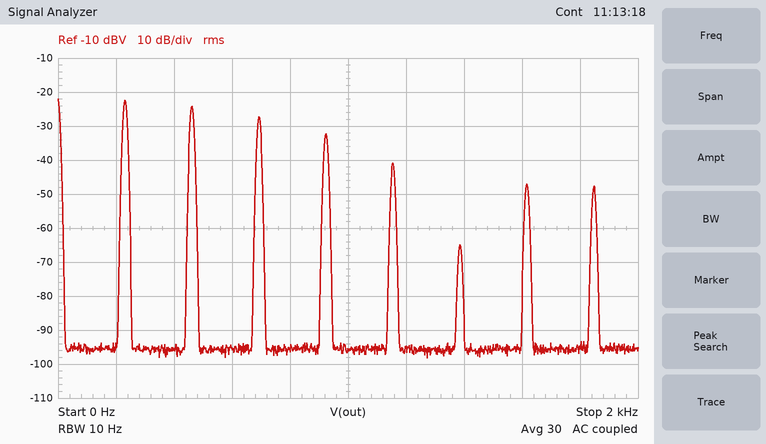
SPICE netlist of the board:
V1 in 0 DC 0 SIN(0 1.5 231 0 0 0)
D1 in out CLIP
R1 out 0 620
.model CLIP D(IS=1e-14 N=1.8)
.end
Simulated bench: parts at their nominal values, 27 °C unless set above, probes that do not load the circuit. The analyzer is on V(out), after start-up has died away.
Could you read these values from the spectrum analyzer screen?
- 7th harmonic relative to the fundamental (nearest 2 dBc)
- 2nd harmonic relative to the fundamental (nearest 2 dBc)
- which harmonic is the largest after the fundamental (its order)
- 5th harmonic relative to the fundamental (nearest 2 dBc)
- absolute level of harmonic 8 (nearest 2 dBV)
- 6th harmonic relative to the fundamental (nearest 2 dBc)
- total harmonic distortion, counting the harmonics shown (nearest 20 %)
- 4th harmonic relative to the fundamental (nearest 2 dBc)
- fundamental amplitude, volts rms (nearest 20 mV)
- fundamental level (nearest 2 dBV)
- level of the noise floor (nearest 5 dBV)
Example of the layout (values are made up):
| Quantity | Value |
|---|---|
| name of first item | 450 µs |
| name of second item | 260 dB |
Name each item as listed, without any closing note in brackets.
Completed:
| Quantity | Value |
|---|---|
| 7th harmonic relative to the fundamental | -24 dBc |
| 2nd harmonic relative to the fundamental | -2 dBc |
| which harmonic is the largest after the fundamental | 2 |
| 5th harmonic relative to the fundamental | -18 dBc |
| absolute level of harmonic 8 | -48 dBV |
| 6th harmonic relative to the fundamental | -42 dBc |
| total harmonic distortion, counting the harmonics shown | 100 % |
| 4th harmonic relative to the fundamental | -10 dBc |
| fundamental amplitude, volts rms | 80 mV |
| fundamental level | -22 dBV |
| level of the noise floor | -95 dBV |
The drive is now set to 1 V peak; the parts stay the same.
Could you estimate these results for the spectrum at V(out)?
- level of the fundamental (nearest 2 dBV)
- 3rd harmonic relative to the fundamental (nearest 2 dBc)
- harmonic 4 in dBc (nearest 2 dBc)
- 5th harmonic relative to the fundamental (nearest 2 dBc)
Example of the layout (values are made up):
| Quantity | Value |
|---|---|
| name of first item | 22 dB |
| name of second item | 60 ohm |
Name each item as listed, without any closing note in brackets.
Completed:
| Quantity | Value |
|---|---|
| level of the fundamental | -58 dBV |
| 3rd harmonic relative to the fundamental | -2 dBc |
| harmonic 4 in dBc | -4 dBc |
| 5th harmonic relative to the fundamental | -6 dBc |
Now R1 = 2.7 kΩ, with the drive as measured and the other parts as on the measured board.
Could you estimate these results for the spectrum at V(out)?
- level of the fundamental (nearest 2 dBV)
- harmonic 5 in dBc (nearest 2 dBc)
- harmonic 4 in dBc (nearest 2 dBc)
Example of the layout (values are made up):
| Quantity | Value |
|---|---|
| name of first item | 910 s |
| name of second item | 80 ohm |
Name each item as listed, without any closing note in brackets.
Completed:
| Quantity | Value |
|---|---|
| level of the fundamental | -20 dBV |
| harmonic 5 in dBc | -24 dBc |
| harmonic 4 in dBc | -12 dBc |
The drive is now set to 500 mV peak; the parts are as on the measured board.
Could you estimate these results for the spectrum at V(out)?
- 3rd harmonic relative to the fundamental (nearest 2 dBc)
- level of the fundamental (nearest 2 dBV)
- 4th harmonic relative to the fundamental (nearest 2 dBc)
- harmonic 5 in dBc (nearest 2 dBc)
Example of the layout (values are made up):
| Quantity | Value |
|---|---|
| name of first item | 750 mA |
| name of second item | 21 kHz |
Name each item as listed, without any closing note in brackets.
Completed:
| Quantity | Value |
|---|---|
| 3rd harmonic relative to the fundamental | -4 dBc |
| level of the fundamental | -146 dBV |
| 4th harmonic relative to the fundamental | -6 dBc |
| harmonic 5 in dBc | -10 dBc |
